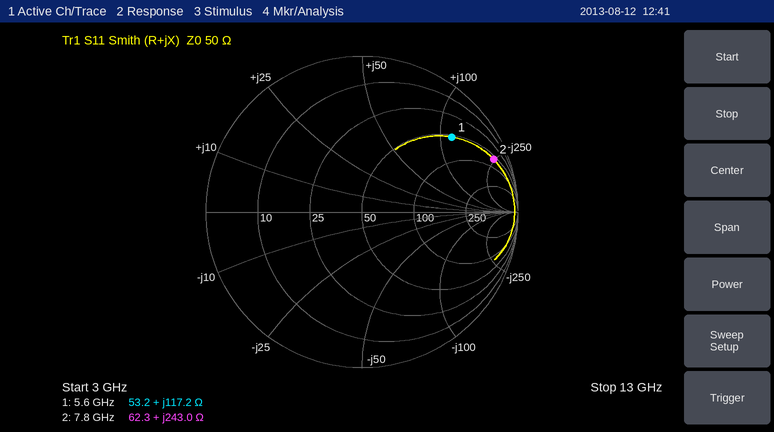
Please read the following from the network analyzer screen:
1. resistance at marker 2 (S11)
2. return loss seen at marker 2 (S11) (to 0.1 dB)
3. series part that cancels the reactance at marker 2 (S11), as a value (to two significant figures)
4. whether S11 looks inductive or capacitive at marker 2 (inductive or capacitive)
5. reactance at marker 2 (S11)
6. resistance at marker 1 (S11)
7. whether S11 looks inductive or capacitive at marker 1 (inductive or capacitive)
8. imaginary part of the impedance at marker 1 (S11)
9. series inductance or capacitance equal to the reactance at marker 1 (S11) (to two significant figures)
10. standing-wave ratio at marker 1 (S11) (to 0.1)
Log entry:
62.3 Ω
0.8 dB
84 fF
inductive
+243.0 Ω
53.2 Ω
inductive
+117.2 Ω
3.3 nH
7.0
